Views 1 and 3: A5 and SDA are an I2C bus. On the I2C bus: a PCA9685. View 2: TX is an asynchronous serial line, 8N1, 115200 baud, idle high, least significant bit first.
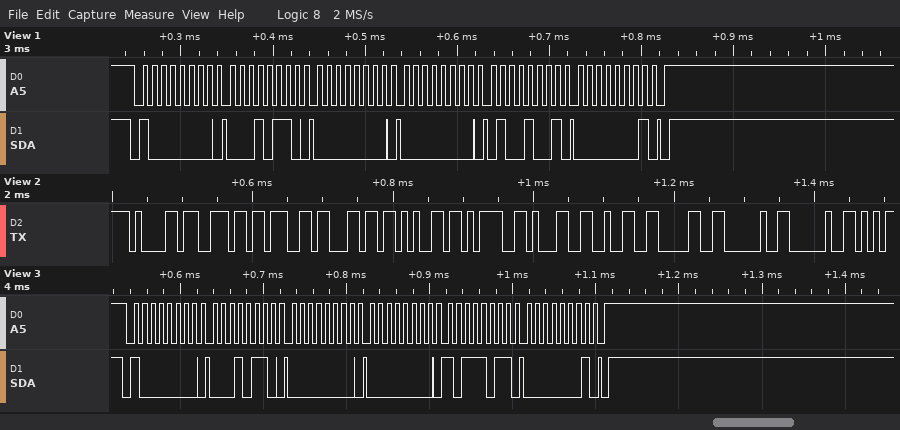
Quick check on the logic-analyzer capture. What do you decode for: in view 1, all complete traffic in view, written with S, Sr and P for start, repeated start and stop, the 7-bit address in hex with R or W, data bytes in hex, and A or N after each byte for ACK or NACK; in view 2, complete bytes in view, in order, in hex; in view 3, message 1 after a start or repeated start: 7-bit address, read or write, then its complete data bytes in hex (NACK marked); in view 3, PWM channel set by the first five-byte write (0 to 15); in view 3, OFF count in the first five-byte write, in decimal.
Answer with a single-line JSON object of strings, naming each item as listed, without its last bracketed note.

{"in view 1, all complete traffic in view, written with S, Sr and P for start, repeated start and stop, the 7-bit address in hex with R or W, data bytes in hex, and A or N after each byte for ACK or NACK": "S 40W A 16 A 00 A 00 A 49 A 01 A P", "in view 2, complete bytes in view, in order, in hex": "61 6E 67 6C 65 3D 31 32 30 20 20", "in view 3, message 1 after a start or repeated start: 7-bit address, read or write, then its complete data bytes in hex": "0x40 write: 16 00 00 BB 01", "in view 3, PWM channel set by the first five-byte write": "4", "in view 3, OFF count in the first five-byte write, in decimal": "443"}
